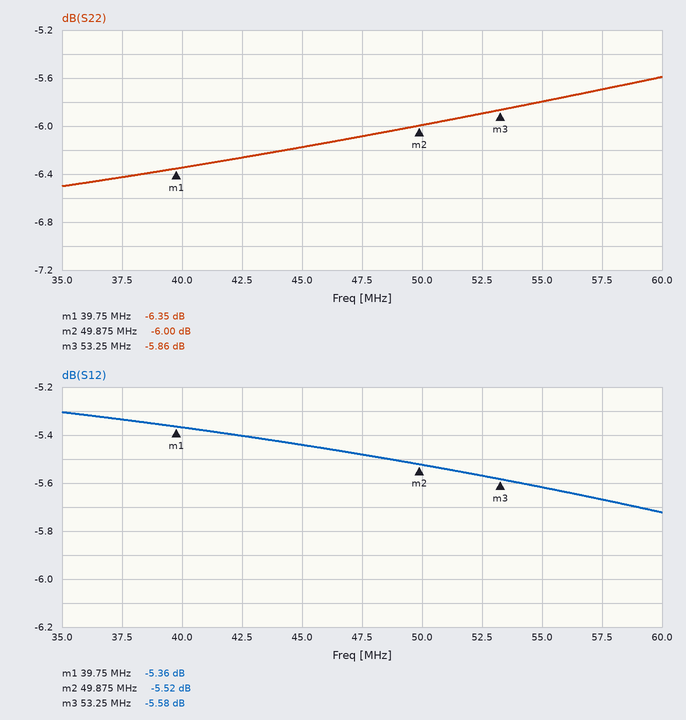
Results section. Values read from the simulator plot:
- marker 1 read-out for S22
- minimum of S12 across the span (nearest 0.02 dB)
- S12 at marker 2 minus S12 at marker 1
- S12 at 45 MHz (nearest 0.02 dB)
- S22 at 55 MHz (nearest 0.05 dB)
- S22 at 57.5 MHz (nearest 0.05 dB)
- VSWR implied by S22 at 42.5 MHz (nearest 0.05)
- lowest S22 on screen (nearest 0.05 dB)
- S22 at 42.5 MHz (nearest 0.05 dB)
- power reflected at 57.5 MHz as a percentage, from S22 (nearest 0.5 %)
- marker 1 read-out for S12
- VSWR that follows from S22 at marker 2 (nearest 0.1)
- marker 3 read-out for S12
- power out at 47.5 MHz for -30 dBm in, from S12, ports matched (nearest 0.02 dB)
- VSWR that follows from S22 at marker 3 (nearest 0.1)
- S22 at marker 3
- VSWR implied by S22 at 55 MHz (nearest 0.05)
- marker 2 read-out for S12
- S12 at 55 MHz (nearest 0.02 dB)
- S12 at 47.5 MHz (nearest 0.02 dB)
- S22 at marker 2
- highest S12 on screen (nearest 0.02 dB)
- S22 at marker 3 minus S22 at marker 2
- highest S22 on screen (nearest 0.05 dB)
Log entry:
-6.35 dB
-5.72 dB
-0.16 dB
-5.44 dB
-5.80 dB
-5.70 dB
2.90
-6.50 dB
-6.25 dB
27.0 %
-5.36 dB
3.0
-5.58 dB
-35.48 dBm
3.1
-5.86 dB
3.10
-5.52 dB
-5.62 dB
-5.48 dB
-6.00 dB
-5.30 dB
0.14 dB
-5.60 dB
